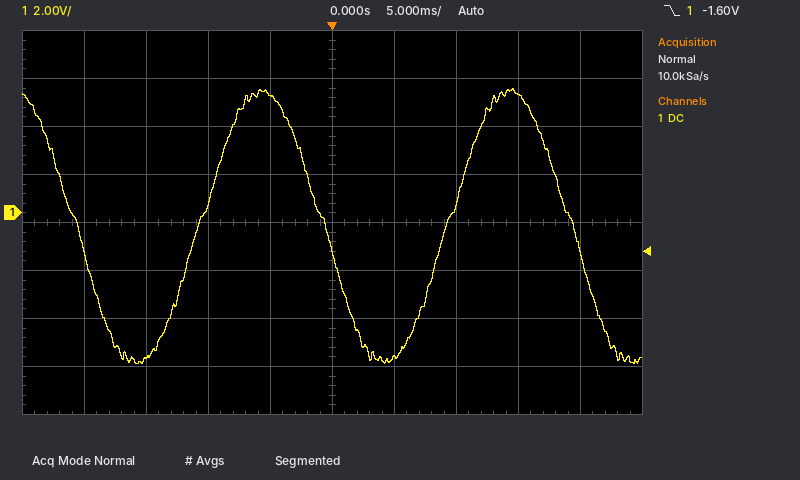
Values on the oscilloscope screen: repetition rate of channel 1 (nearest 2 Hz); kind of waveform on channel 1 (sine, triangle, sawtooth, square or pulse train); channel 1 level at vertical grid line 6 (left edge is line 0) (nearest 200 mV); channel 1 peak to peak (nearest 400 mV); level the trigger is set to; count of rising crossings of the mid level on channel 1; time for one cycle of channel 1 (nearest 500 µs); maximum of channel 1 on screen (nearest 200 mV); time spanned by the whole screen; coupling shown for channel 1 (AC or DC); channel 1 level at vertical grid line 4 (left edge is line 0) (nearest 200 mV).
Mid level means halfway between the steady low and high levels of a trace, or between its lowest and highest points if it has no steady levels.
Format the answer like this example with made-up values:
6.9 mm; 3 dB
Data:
50 Hz; sine; -6.0 V; 11.6 V; -1.60 V; 2; 20.0 ms; 5.2 V; 50 ms; DC; 5.0 V
